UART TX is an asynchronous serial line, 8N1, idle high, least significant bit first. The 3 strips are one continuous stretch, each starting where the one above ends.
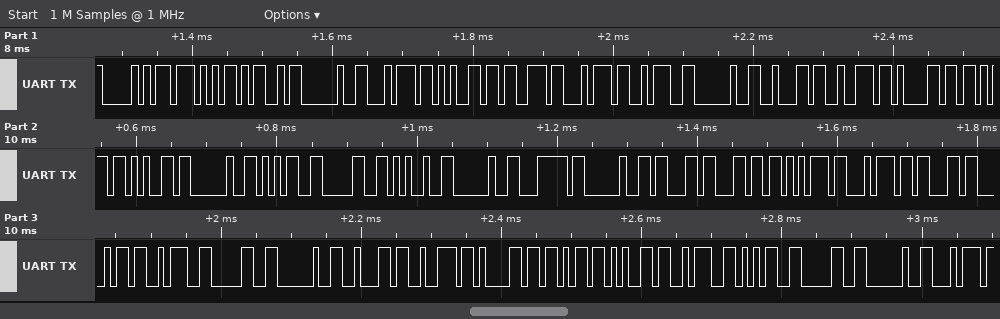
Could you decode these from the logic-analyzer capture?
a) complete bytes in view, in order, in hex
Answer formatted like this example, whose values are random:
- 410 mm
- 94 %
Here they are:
- 50 57 4D 20 74 65 73 74 3A 20 62 72 61 6B 65 20 35 30 25 20 7C 20 63 6C 75 74 63 68 3A 30 20 62 72 61 6B 65 3A 35 30 20 74
